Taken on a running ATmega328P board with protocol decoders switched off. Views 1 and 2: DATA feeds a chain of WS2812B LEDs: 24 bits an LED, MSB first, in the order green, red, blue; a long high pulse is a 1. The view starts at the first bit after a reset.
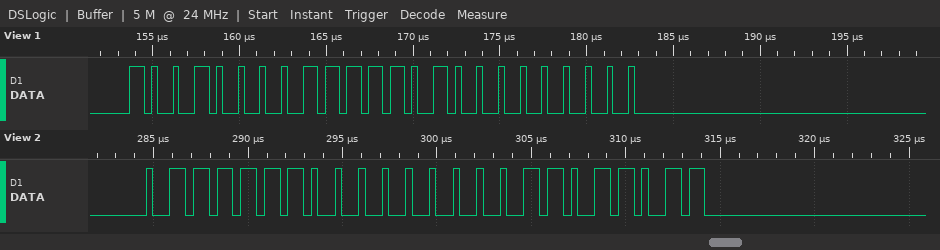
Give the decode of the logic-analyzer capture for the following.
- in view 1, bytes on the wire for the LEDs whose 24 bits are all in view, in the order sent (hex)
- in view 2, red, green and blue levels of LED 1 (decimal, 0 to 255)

90 FA 00
0, 126, 219
